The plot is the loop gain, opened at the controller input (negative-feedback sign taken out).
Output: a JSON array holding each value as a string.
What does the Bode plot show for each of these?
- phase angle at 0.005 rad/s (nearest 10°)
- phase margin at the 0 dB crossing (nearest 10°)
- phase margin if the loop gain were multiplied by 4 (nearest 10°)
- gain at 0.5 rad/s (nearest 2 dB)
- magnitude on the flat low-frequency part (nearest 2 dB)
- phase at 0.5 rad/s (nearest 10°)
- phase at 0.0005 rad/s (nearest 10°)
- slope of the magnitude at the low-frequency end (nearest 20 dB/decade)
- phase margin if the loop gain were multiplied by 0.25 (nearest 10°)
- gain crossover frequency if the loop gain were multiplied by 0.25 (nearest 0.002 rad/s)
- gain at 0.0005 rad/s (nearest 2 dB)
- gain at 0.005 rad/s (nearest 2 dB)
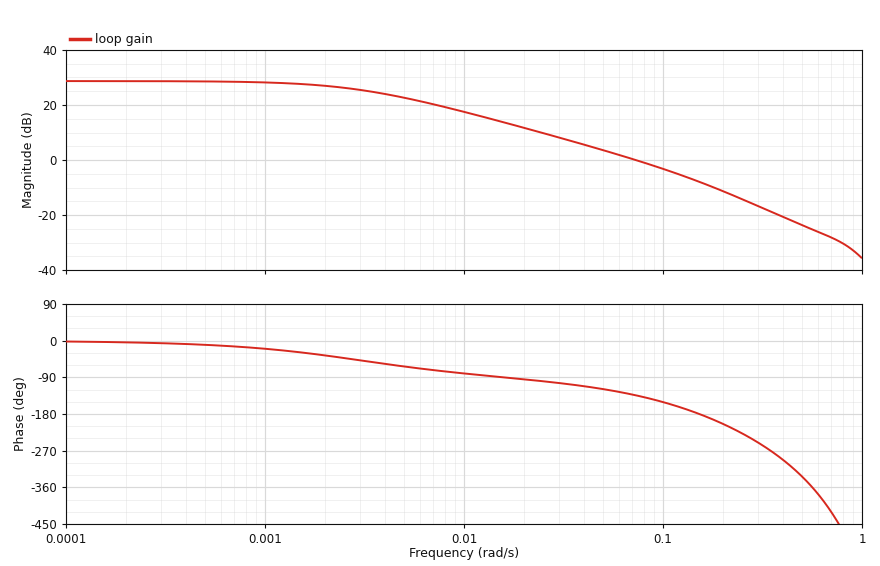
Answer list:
["-60°", "50°", "-30°", "-24 dB", "28 dB", "-330°", "-10°", "0 dB/decade", "90°", "0.020 rad/s", "28 dB", "22 dB"]
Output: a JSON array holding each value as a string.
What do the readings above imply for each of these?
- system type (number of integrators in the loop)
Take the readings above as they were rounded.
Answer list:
["0"]
